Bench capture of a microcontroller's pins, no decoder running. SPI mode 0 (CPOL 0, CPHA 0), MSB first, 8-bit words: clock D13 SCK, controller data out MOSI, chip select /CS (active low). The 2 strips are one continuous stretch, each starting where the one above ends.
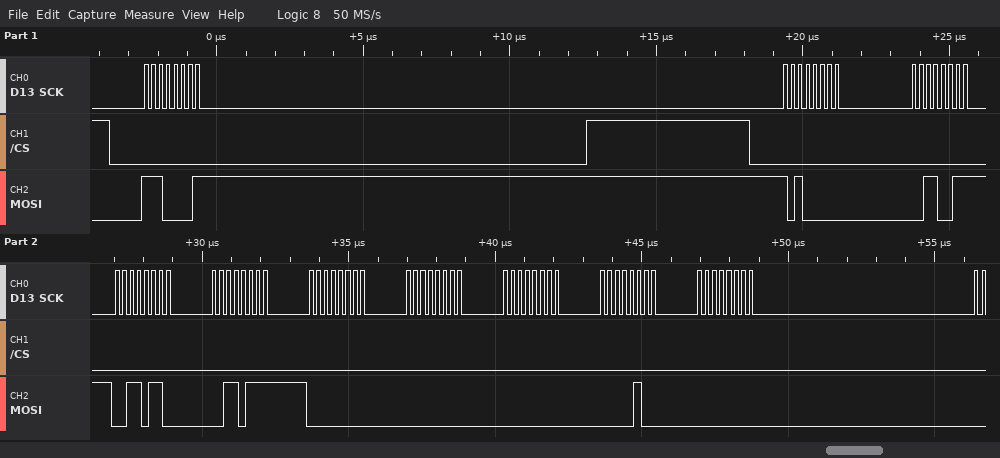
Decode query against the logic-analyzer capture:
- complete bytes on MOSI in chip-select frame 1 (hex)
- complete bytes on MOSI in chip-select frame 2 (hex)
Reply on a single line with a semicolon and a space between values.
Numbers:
0xE1; 0xA0 0x33 0x36 0x37 0x00 0x00 0x00 0x04 0x00
